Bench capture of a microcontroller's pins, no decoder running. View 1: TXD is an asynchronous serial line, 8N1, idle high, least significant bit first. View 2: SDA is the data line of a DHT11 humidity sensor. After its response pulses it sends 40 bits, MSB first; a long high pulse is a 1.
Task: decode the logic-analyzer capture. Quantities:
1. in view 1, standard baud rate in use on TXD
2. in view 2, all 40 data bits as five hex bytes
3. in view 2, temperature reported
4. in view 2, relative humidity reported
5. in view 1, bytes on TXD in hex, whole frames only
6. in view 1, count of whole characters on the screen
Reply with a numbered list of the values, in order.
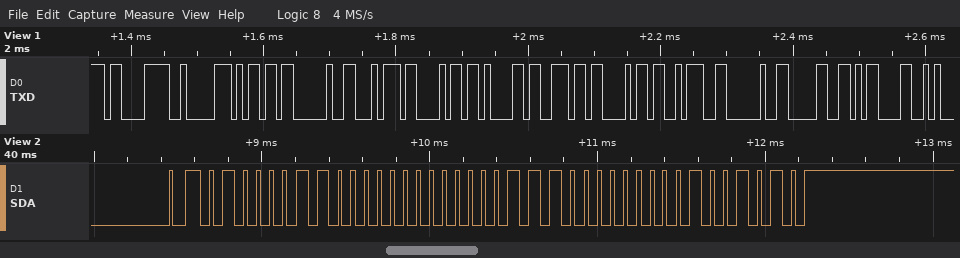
1. 115200 baud
2. 43 00 07 00 4A
3. 7.0 °C
4. 67 %
5. C3 82 6D 20 74 68 61 6E 68 3A 20 30 0D
6. 13
